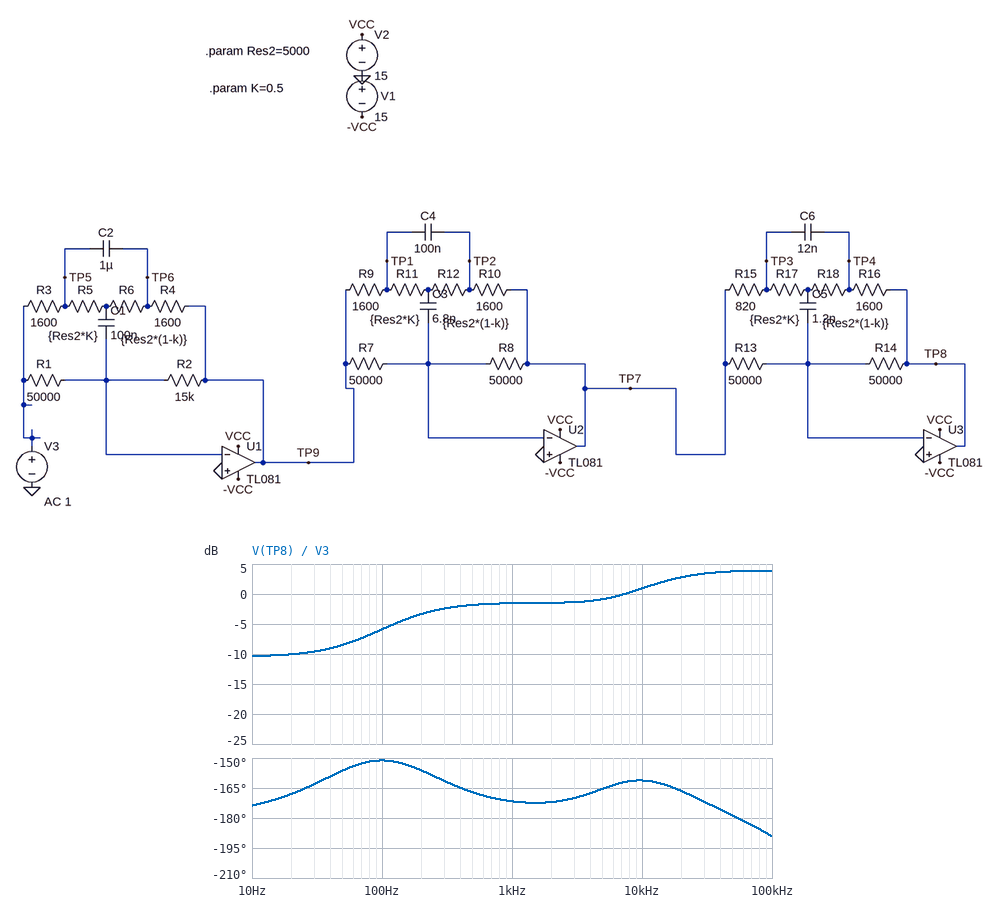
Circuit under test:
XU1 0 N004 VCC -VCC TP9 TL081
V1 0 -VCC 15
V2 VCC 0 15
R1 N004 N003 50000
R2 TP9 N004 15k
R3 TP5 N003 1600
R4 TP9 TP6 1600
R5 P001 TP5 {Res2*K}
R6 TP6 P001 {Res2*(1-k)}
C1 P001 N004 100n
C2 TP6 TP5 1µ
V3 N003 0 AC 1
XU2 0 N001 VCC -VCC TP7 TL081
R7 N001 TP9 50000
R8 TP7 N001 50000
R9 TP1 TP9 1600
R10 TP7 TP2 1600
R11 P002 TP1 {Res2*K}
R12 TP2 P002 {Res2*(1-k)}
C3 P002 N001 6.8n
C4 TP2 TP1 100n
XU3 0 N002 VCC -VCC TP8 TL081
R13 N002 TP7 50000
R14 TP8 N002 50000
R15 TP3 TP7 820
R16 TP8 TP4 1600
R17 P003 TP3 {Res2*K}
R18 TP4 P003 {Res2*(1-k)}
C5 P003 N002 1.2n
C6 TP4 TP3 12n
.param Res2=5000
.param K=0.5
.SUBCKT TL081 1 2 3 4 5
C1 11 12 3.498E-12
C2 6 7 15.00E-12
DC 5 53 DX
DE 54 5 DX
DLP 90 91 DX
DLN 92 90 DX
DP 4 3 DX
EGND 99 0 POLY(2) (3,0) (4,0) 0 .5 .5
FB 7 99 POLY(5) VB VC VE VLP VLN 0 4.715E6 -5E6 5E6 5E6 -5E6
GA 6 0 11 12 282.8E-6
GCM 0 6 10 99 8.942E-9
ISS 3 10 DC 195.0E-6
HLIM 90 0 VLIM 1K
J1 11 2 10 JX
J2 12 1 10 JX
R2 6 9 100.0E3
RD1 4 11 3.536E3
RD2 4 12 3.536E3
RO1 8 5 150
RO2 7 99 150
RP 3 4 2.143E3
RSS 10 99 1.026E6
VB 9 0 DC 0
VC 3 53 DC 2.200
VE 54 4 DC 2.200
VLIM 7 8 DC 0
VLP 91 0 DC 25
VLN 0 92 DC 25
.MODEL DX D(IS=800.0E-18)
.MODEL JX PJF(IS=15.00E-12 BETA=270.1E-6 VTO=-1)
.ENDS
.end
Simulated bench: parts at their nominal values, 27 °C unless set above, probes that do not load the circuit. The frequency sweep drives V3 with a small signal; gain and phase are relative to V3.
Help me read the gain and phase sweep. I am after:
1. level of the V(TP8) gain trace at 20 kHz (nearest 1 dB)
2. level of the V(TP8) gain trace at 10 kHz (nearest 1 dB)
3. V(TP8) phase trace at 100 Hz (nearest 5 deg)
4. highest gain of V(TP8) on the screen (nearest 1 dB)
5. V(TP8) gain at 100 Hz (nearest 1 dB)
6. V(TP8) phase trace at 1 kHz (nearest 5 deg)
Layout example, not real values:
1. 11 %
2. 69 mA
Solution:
1. 3 dB
2. 1 dB
3. -150 deg
4. 4 dB
5. -6 dB
6. -170 deg
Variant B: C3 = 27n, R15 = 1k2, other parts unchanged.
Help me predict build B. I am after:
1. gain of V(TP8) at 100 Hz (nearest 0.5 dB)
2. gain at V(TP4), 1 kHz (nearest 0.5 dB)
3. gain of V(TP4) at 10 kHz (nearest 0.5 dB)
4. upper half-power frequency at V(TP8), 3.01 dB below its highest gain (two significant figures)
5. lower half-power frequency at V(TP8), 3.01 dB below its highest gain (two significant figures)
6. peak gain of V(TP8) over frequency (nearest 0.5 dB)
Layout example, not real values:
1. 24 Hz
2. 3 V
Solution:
1. -6.0 dB
2. -6.0 dB
3. -10.5 dB
4. 1.0 MHz
5. 360 Hz
6. 1.0 dB
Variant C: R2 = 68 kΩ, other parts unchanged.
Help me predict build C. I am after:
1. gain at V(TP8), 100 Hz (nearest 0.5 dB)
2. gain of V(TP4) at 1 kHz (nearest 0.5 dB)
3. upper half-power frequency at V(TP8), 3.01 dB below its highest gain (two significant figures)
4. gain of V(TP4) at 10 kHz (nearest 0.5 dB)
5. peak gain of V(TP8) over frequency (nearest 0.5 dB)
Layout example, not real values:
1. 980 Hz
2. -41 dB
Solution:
1. 0.5 dB
2. -5.0 dB
3. 850 kHz
4. -8.5 dB
5. 5.5 dB
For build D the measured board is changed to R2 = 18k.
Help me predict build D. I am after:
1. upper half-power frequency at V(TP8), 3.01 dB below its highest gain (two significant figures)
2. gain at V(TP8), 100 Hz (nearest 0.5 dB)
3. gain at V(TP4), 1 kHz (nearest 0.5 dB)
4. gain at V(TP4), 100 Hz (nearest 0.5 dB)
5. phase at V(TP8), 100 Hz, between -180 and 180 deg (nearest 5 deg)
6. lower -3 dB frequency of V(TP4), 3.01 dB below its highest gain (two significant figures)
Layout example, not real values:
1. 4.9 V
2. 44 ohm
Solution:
1. 870 kHz
2. -4.5 dB
3. -6.0 dB
4. -9.5 dB
5. -155 deg
6. 110 Hz
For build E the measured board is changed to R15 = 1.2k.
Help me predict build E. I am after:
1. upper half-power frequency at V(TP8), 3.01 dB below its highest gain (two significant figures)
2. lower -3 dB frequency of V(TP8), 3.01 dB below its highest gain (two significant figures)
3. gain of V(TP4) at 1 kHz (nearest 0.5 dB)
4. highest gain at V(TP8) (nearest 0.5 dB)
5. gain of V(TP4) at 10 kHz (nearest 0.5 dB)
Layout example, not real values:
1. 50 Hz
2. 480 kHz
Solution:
1. 1.0 MHz
2. 360 Hz
3. -6.0 dB
4. 1.0 dB
5. -10.5 dB
